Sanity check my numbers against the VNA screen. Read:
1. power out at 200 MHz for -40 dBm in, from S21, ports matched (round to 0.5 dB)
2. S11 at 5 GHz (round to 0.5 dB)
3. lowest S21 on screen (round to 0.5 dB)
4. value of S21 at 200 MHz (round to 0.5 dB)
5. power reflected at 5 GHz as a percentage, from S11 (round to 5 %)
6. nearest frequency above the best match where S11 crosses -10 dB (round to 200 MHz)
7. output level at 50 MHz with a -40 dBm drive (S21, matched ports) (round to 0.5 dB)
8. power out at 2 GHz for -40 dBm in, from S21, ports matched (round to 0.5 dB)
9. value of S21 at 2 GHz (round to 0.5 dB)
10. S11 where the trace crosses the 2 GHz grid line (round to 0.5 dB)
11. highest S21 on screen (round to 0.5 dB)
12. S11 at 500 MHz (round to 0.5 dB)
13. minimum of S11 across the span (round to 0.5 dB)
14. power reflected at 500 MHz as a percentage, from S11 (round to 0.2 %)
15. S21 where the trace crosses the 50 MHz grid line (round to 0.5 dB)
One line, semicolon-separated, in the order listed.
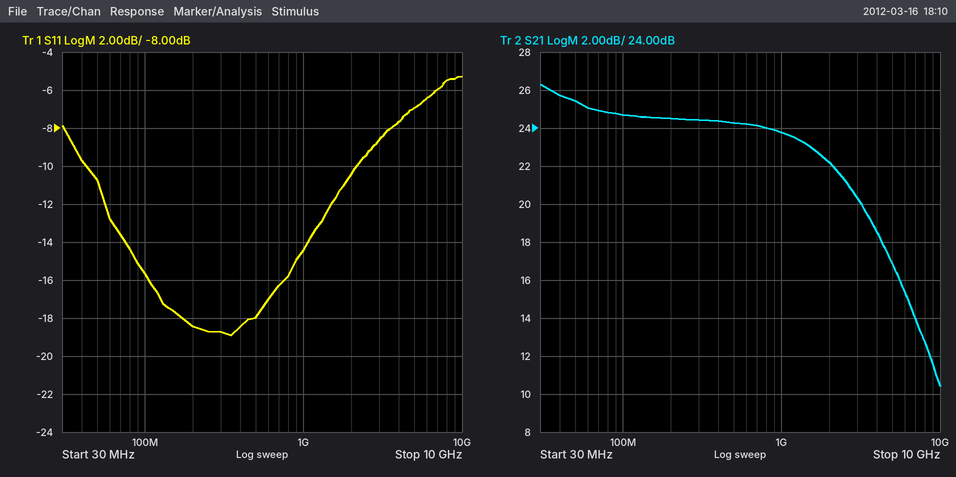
-15.5 dBm; -7.0 dB; 10.5 dB; 24.5 dB; 20 %; 2.2 GHz; -14.5 dBm; -18.0 dBm; 22.0 dB; -10.5 dB; 26.5 dB; -18.0 dB; -19.0 dB; 1.6 %; 25.5 dB
